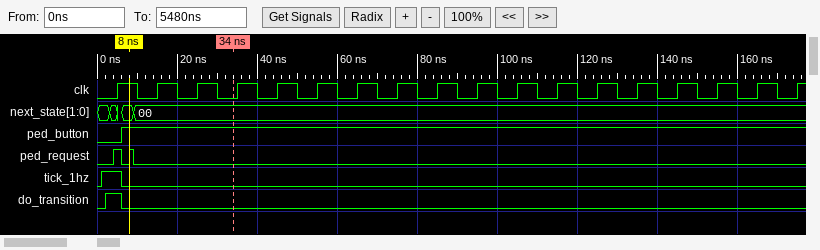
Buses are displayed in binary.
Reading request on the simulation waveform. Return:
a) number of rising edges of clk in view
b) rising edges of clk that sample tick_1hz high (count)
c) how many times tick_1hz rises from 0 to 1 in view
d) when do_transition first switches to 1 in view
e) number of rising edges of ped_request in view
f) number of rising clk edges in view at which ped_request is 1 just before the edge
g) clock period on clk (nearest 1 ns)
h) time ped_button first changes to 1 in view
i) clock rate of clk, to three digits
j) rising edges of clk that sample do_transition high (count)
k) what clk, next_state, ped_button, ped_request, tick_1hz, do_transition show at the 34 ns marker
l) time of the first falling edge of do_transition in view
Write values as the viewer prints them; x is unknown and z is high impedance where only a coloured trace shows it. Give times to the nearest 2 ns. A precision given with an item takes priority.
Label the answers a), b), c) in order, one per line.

a) 18
b) 1
c) 1
d) 2 ns
e) 2
f) 1
g) 10 ns
h) 6 ns
i) 100 MHz
j) 1
k) clk=0, next_state=00, ped_button=1, ped_request=0, tick_1hz=0, do_transition=0
l) 6 ns
